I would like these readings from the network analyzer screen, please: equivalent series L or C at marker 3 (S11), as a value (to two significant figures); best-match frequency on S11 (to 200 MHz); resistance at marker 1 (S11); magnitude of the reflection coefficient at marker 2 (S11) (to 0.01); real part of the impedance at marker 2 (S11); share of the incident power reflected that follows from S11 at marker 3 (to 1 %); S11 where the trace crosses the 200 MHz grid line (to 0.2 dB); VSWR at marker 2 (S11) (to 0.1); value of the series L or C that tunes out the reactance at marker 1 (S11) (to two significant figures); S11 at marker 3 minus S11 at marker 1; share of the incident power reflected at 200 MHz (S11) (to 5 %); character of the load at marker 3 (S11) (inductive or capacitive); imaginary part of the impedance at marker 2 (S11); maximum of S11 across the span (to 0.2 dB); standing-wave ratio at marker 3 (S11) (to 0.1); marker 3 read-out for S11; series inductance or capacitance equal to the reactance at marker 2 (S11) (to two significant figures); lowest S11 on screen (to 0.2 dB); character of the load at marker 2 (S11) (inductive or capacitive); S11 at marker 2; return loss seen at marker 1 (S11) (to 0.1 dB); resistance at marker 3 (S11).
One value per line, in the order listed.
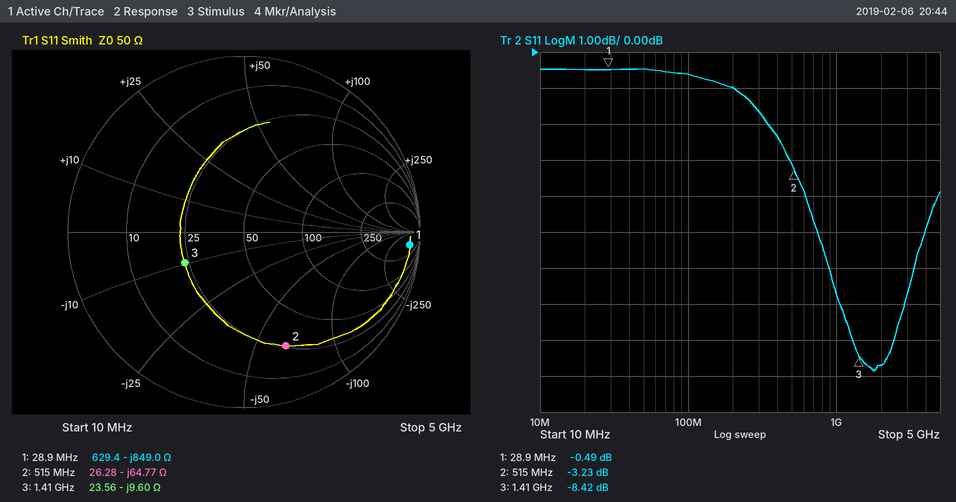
12 pF
1.8 GHz
629.4 Ω
0.69
26.28 Ω
14 %
-1.0 dB
5.4
4.7 µH
-7.93 dB
80 %
capacitive
-64.77 Ω
-0.4 dB
2.2
-8.42 dB
4.8 pF
-8.8 dB
capacitive
-3.23 dB
0.5 dB
23.56 Ω
